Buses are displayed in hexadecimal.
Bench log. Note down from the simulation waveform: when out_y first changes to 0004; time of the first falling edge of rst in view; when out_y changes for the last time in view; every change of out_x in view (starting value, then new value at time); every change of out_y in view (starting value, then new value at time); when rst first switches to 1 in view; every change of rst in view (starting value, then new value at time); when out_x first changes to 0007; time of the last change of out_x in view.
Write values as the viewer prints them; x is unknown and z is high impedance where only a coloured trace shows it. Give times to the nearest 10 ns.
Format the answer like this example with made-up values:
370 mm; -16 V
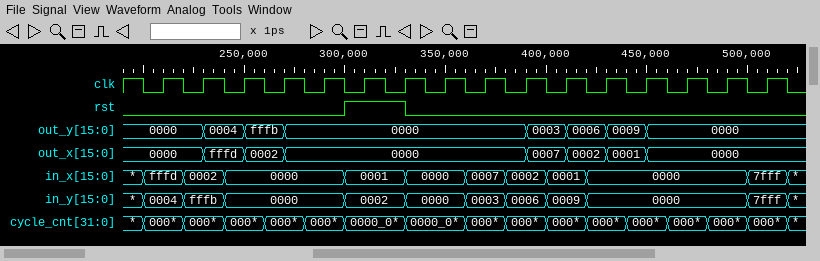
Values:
230 ns; 330 ns; 450 ns; 0000, fffd at 230 ns, 0002 at 250 ns, 0000 at 270 ns, 0007 at 390 ns, 0002 at 410 ns, 0001 at 430 ns, 0000 at 450 ns; 0000, 0004 at 230 ns, fffb at 250 ns, 0000 at 270 ns, 0003 at 390 ns, 0006 at 410 ns, 0009 at 430 ns, 0000 at 450 ns; 300 ns; 0, 1 at 300 ns, 0 at 330 ns; 390 ns; 450 ns
